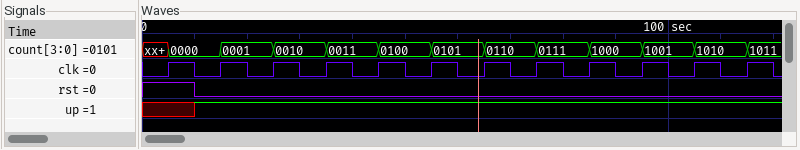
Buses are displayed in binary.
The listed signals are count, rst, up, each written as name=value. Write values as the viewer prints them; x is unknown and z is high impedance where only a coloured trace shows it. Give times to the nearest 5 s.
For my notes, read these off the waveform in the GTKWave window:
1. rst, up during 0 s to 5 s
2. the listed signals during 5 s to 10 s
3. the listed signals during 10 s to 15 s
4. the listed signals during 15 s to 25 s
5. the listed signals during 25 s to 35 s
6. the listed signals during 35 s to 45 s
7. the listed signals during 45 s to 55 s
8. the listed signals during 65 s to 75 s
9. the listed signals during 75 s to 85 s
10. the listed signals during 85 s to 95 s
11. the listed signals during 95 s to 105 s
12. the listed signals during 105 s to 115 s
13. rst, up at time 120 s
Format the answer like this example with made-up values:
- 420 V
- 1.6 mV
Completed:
- rst=1, up=x
- count=0000, rst=1, up=x
- count=0000, rst=0, up=1
- count=0001, rst=0, up=1
- count=0010, rst=0, up=1
- count=0011, rst=0, up=1
- count=0100, rst=0, up=1
- count=0110, rst=0, up=1
- count=0111, rst=0, up=1
- count=1000, rst=0, up=1
- count=1001, rst=0, up=1
- count=1010, rst=0, up=1
- rst=0, up=1
